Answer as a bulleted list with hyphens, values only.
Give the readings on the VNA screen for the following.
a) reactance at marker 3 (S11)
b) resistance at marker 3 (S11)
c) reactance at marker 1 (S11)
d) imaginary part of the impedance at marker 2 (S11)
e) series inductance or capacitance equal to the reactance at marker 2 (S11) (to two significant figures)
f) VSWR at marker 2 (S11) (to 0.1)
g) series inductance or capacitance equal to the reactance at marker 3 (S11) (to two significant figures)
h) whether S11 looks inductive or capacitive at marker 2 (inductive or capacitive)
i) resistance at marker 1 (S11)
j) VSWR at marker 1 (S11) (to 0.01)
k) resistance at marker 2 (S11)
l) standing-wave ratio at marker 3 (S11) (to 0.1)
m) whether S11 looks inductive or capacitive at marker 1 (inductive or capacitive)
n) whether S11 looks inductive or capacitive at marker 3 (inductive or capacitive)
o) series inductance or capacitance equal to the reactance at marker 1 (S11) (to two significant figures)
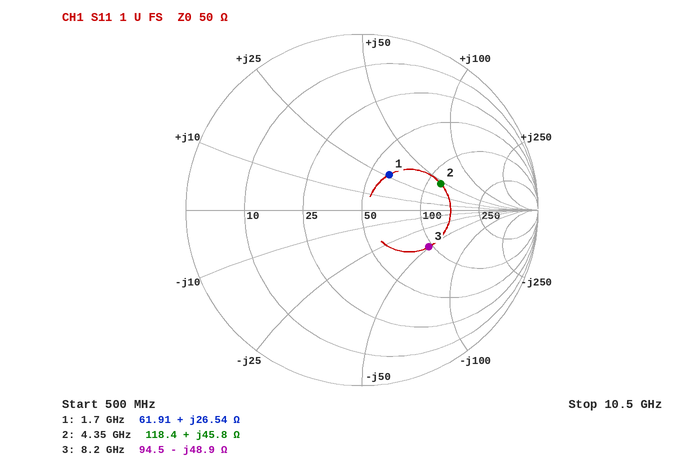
- -48.9 Ω
- 94.5 Ω
- +26.54 Ω
- +45.8 Ω
- 1.7 nH
- 2.8
- 400 fF
- inductive
- 61.91 Ω
- 1.68
- 118.4 Ω
- 2.5
- inductive
- capacitive
- 2.5 nH
